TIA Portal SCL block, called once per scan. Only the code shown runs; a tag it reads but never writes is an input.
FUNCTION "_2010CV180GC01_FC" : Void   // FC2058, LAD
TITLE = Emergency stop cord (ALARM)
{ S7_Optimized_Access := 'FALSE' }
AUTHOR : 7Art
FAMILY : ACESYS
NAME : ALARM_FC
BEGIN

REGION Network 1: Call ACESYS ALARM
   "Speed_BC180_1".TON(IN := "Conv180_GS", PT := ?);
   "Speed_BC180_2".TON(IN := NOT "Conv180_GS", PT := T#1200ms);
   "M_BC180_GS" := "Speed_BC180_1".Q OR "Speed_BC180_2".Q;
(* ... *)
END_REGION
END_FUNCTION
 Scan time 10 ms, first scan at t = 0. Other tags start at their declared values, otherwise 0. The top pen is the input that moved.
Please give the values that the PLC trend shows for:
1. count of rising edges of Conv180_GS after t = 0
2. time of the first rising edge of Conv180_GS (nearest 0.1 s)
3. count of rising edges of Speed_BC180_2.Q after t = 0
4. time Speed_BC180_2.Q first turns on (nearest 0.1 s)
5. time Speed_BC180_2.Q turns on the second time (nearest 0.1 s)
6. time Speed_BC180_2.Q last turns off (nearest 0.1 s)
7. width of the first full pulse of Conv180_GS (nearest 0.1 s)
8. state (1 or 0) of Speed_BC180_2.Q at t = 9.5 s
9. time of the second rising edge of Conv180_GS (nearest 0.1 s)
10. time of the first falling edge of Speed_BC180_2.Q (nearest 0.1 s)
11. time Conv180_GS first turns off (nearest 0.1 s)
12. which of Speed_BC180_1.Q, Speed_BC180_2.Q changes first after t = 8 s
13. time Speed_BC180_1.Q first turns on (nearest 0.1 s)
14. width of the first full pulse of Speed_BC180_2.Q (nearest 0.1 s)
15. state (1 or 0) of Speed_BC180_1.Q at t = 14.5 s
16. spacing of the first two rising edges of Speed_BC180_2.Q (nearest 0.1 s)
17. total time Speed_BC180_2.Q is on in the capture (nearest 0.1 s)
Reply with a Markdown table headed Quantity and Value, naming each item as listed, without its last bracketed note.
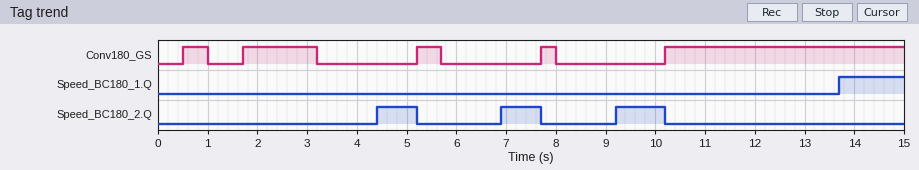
| Quantity | Value |
|---|---|
| count of rising edges of Conv180_GS after t = 0 | 5 |
| time of the first rising edge of Conv180_GS | 0.5 s |
| count of rising edges of Speed_BC180_2.Q after t = 0 | 3 |
| time Speed_BC180_2.Q first turns on | 4.4 s |
| time Speed_BC180_2.Q turns on the second time | 6.9 s |
| time Speed_BC180_2.Q last turns off | 10.2 s |
| width of the first full pulse of Conv180_GS | 0.5 s |
| state (1 or 0) of Speed_BC180_2.Q at t = 9.5 s | 1 |
| time of the second rising edge of Conv180_GS | 1.7 s |
| time of the first falling edge of Speed_BC180_2.Q | 5.2 s |
| time Conv180_GS first turns off | 1.0 s |
| which of Speed_BC180_1.Q, Speed_BC180_2.Q changes first after t = 8 s | Speed_BC180_2.Q |
| time Speed_BC180_1.Q first turns on | 13.7 s |
| width of the first full pulse of Speed_BC180_2.Q | 0.8 s |
| state (1 or 0) of Speed_BC180_1.Q at t = 14.5 s | 1 |
| spacing of the first two rising edges of Speed_BC180_2.Q | 2.5 s |
| total time Speed_BC180_2.Q is on in the capture | 2.6 s |
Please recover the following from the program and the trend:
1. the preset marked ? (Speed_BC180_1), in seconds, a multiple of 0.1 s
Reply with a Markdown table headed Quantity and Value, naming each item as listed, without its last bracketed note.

| Quantity | Value |
|---|---|
| the preset marked ? (Speed_BC180_1), in seconds, a multiple of 0.1 s | 3.5 s |
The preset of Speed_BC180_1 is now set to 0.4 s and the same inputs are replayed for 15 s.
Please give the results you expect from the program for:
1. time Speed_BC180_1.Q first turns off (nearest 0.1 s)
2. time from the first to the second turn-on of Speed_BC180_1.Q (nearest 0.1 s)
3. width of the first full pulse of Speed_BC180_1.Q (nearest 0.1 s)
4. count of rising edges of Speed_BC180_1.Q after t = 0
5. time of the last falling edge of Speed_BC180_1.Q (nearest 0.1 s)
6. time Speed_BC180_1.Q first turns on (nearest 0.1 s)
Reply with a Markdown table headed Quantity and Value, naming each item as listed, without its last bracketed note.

| Quantity | Value |
|---|---|
| time Speed_BC180_1.Q first turns off | 1.0 s |
| time from the first to the second turn-on of Speed_BC180_1.Q | 1.2 s |
| width of the first full pulse of Speed_BC180_1.Q | 0.1 s |
| count of rising edges of Speed_BC180_1.Q after t = 0 | 4 |
| time of the last falling edge of Speed_BC180_1.Q | 5.7 s |
| time Speed_BC180_1.Q first turns on | 0.9 s |
